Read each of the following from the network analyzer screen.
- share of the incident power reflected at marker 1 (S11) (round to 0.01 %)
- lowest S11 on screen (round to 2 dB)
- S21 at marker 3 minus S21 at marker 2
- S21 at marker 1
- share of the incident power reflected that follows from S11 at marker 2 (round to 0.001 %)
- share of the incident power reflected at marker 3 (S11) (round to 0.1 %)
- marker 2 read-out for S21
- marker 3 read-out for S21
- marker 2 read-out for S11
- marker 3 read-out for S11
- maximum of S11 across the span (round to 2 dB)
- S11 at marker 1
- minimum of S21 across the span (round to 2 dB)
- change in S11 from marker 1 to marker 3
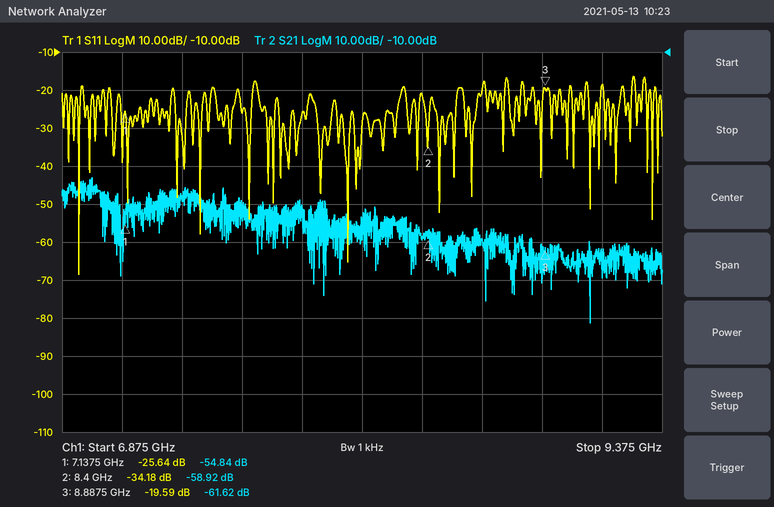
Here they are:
0.27 %
-68 dB
-2.70 dB
-54.84 dB
0.038 %
1.1 %
-58.92 dB
-61.62 dB
-34.18 dB
-19.59 dB
-16 dB
-25.64 dB
-82 dB
6.05 dB
